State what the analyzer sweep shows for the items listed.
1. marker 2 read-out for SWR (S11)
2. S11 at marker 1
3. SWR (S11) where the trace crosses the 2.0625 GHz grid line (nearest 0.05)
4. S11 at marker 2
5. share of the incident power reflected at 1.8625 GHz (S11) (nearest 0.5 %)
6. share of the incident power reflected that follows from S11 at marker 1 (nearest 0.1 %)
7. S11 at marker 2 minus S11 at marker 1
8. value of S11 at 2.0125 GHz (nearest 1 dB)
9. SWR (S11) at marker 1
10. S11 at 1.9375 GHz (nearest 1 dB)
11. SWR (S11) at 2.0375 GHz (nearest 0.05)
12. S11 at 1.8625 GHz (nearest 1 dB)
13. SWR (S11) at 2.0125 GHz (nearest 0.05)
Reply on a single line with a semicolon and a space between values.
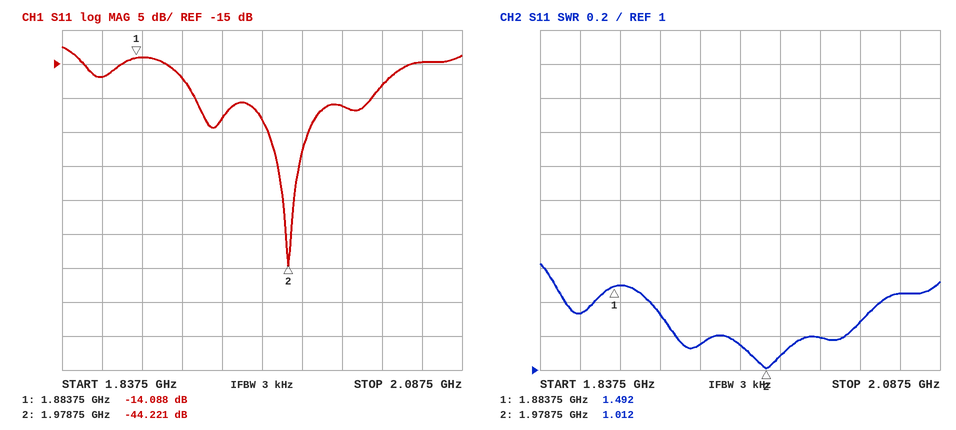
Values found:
1.012; -14.088 dB; 1.45; -44.221 dB; 2.0 %; 3.9 %; -30.133 dB; -21 dB; 1.492; -23 dB; 1.30; -17 dB; 1.20
